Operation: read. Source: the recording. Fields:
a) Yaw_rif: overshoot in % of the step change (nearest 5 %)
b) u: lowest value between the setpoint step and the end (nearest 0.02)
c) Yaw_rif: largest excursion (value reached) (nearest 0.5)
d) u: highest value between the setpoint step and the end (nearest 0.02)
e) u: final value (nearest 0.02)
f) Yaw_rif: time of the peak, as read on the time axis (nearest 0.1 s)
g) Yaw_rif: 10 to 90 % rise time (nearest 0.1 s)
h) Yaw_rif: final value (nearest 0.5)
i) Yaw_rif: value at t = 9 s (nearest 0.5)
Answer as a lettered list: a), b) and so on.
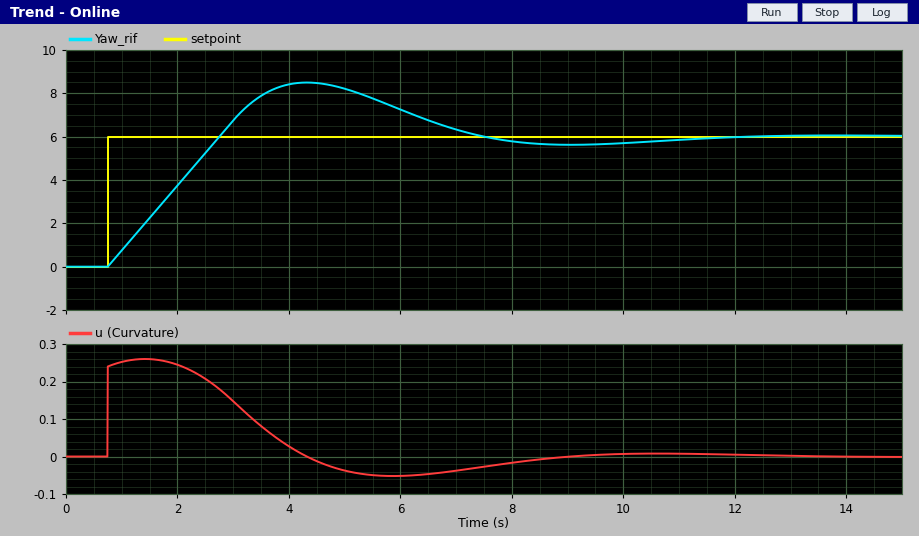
a) 40 %
b) -0.06
c) 8.5
d) 0.26
e) 0.00
f) 4.3 s
g) 1.6 s
h) 6.0
i) 5.5
